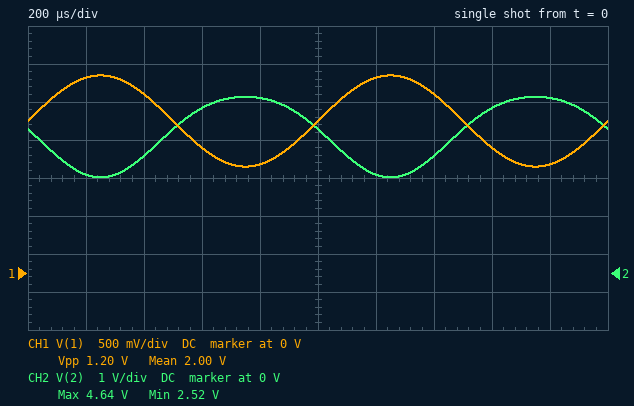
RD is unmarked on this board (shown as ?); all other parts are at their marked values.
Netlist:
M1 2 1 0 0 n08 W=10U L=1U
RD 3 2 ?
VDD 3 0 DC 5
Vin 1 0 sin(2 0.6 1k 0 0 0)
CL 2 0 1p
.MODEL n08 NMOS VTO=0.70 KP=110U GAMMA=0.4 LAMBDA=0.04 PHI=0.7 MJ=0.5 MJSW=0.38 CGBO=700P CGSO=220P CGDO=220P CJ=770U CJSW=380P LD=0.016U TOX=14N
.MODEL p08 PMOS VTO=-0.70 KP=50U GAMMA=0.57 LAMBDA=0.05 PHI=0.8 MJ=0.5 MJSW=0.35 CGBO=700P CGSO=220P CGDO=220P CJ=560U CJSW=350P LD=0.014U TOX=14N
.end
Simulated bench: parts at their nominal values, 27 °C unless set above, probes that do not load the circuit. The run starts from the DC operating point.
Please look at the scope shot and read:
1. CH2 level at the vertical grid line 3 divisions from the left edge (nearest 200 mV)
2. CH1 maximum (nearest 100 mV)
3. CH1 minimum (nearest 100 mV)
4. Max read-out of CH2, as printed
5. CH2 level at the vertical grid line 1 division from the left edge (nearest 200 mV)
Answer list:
4.4 V
2.6 V
1.4 V
4.64 V
2.6 V
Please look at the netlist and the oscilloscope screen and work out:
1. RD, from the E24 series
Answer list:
1.1 kΩ
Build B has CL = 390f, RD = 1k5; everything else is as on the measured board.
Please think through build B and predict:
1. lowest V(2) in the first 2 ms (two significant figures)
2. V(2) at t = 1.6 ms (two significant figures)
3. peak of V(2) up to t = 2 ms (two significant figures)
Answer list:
1.7 V
4.1 V
4.5 V
